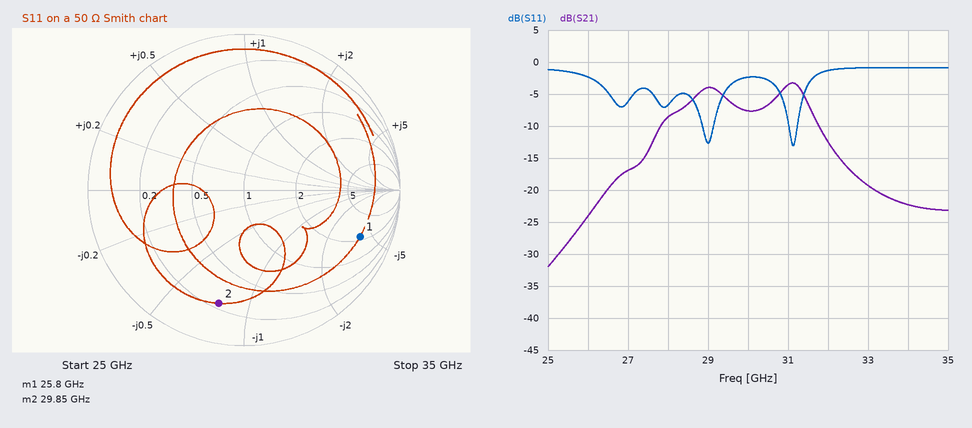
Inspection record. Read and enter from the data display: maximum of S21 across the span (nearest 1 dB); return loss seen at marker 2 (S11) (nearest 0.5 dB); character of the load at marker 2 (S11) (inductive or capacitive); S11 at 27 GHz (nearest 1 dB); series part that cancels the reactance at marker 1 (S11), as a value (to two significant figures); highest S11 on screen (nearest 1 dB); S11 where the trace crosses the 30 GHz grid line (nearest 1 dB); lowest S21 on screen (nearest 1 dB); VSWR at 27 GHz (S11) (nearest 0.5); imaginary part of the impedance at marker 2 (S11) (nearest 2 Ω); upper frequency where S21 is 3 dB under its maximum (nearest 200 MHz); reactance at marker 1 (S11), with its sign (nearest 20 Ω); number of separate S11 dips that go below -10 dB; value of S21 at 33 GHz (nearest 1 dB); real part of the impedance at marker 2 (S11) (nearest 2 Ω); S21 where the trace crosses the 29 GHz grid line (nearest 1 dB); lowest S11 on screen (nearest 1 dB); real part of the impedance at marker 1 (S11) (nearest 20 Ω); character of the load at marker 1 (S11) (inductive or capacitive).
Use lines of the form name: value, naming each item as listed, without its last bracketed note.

maximum of S21 across the span: -3 dB
return loss seen at marker 2 (S11): 2.5 dB
character of the load at marker 2 (S11): capacitive
S11 at 27 GHz: -6 dB
series part that cancels the reactance at marker 1 (S11), as a value: 1.2 nH
highest S11 on screen: -1 dB
S11 where the trace crosses the 30 GHz grid line: -2 dB
lowest S21 on screen: -32 dB
VSWR at 27 GHz (S11): 3.0
imaginary part of the impedance at marker 2 (S11): -38 Ω
upper frequency where S21 is 3 dB under its maximum: 31.4 GHz
reactance at marker 1 (S11), with its sign: -200 Ω
number of separate S11 dips that go below -10 dB: 2
value of S21 at 33 GHz: -19 dB
real part of the impedance at marker 2 (S11): 12 Ω
S21 where the trace crosses the 29 GHz grid line: -4 dB
lowest S11 on screen: -13 dB
real part of the impedance at marker 1 (S11): 120 Ω
character of the load at marker 1 (S11): capacitive
